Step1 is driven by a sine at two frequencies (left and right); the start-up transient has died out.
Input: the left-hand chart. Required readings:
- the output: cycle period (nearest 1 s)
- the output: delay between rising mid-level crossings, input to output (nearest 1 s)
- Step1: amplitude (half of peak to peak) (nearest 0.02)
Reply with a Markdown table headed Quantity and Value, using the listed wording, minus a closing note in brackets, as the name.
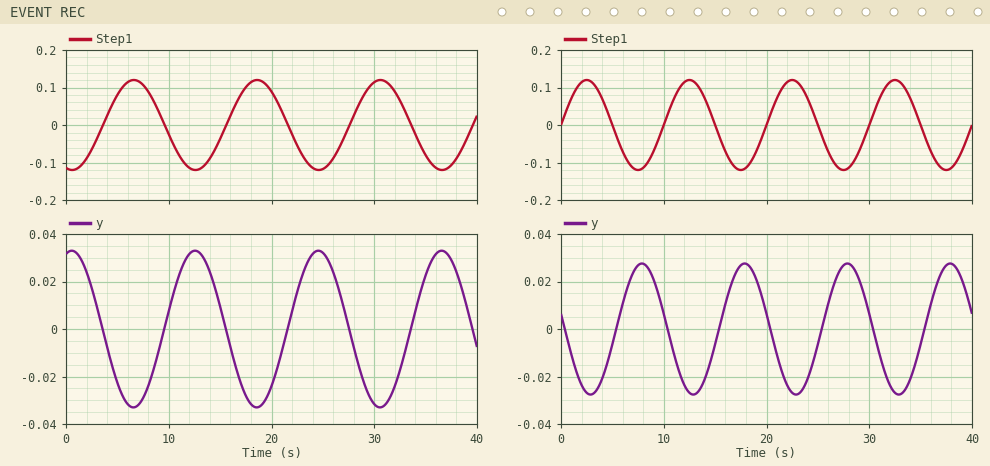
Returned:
| Quantity | Value |
|---|---|
| the output: cycle period | 12 s |
| the output: delay between rising mid-level crossings, input to output | 6 s |
| Step1: amplitude (half of peak to peak) | 0.12 |
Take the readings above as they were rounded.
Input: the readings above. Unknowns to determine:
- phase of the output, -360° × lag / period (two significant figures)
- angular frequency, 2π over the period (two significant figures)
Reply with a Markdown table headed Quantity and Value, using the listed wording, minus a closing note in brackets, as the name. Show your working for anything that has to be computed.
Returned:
| Quantity | Value |
|---|---|
| phase of the output, -360° × lag / period | -360 × 6 / 12 = -180° |
| angular frequency, 2π over the period | 2π / 12 = 0.52 rad/s |
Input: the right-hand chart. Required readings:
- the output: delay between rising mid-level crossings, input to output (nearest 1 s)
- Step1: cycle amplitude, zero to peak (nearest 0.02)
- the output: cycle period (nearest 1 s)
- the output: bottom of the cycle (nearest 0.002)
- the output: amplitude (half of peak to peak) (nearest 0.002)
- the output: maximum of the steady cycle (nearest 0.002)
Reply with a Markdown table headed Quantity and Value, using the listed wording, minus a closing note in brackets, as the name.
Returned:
| Quantity | Value |
|---|---|
| the output: delay between rising mid-level crossings, input to output | 5 s |
| Step1: cycle amplitude, zero to peak | 0.12 |
| the output: cycle period | 10 s |
| the output: bottom of the cycle | -0.028 |
| the output: amplitude (half of peak to peak) | 0.028 |
| the output: maximum of the steady cycle | 0.028 |
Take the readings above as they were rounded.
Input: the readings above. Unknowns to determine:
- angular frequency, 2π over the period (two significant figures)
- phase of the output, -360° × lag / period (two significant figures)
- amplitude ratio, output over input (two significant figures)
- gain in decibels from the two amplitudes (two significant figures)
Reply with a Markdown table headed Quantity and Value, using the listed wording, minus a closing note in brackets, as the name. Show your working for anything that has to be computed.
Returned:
| Quantity | Value |
|---|---|
| angular frequency, 2π over the period | 2π / 10 = 0.63 rad/s |
| phase of the output, -360° × lag / period | -360 × 5 / 10 = -180° |
| amplitude ratio, output over input | 0.028 / 0.12 = 0.23 |
| gain in decibels from the two amplitudes | 20 log10(0.028 / 0.12) = -13 dB |
